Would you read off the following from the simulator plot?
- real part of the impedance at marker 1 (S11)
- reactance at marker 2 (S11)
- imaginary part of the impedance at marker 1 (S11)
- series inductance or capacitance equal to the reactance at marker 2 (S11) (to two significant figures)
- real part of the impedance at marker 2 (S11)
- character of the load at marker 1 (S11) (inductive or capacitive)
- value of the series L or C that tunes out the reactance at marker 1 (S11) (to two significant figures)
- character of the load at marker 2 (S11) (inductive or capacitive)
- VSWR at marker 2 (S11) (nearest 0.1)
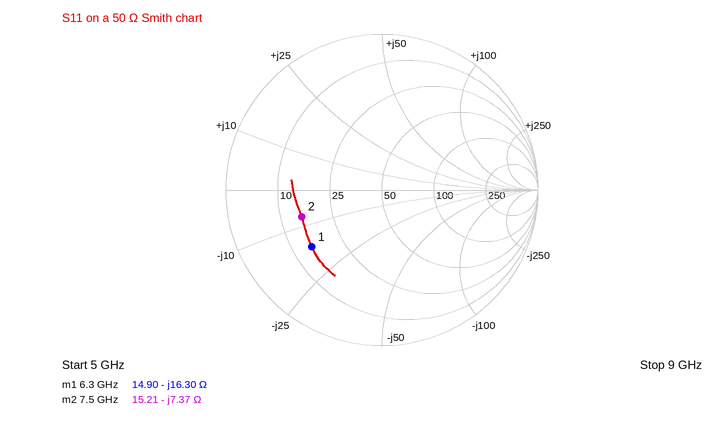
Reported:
14.90 Ω
-7.37 Ω
-16.30 Ω
2.9 pF
15.21 Ω
capacitive
410 pH
capacitive
3.4
